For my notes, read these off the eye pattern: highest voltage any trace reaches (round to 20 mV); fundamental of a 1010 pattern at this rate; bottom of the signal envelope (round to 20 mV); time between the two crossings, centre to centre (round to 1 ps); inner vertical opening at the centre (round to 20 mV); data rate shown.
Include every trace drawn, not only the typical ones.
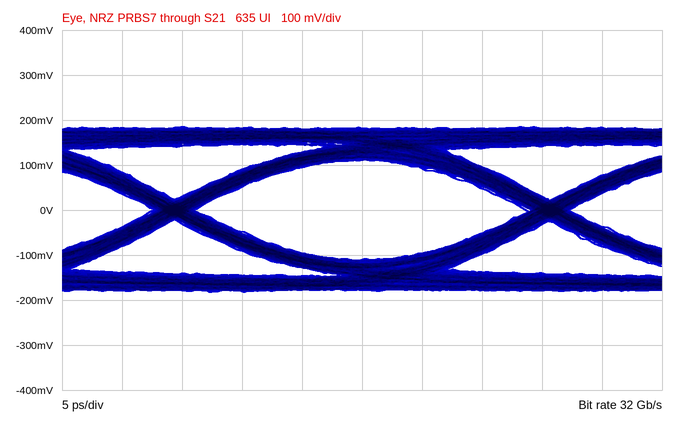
180 mV
16 GHz
-180 mV
31 ps
220 mV
32 Gb/s
